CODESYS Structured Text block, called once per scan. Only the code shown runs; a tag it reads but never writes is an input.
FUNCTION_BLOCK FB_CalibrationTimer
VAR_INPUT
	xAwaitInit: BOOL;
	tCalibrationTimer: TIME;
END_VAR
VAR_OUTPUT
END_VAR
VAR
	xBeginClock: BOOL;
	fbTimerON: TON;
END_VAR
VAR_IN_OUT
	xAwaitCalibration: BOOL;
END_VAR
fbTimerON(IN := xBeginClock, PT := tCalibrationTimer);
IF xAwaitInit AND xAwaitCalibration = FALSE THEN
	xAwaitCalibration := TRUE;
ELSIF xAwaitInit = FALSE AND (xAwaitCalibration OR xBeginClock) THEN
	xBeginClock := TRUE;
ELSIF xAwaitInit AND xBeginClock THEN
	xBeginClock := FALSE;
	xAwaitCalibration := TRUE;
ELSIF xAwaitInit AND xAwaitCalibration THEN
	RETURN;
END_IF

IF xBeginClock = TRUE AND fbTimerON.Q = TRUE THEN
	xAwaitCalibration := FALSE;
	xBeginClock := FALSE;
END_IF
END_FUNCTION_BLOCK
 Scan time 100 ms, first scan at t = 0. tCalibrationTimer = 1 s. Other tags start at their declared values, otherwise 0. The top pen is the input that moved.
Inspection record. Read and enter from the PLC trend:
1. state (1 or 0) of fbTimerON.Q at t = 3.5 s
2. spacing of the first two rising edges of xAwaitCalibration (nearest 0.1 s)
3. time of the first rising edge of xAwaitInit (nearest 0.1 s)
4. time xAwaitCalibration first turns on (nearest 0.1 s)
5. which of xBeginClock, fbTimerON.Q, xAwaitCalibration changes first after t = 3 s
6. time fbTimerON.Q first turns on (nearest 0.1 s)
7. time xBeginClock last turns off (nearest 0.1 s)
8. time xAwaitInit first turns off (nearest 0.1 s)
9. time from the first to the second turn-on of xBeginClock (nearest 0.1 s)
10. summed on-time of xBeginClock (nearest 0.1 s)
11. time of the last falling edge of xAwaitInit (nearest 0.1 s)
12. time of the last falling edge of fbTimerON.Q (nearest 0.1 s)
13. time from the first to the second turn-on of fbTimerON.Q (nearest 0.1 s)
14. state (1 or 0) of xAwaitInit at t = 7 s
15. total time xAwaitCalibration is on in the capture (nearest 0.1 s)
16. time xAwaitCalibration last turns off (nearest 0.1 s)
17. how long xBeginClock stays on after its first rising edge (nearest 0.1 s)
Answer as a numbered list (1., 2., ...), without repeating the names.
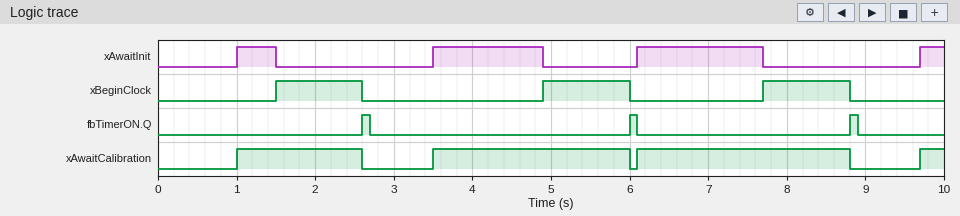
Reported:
1. 0
2. 2.5 s
3. 1.0 s
4. 1.0 s
5. xAwaitCalibration
6. 2.6 s
7. 8.8 s
8. 1.5 s
9. 3.4 s
10. 3.3 s
11. 7.7 s
12. 8.9 s
13. 3.4 s
14. 1
15. 7.1 s
16. 8.8 s
17. 1.1 s
